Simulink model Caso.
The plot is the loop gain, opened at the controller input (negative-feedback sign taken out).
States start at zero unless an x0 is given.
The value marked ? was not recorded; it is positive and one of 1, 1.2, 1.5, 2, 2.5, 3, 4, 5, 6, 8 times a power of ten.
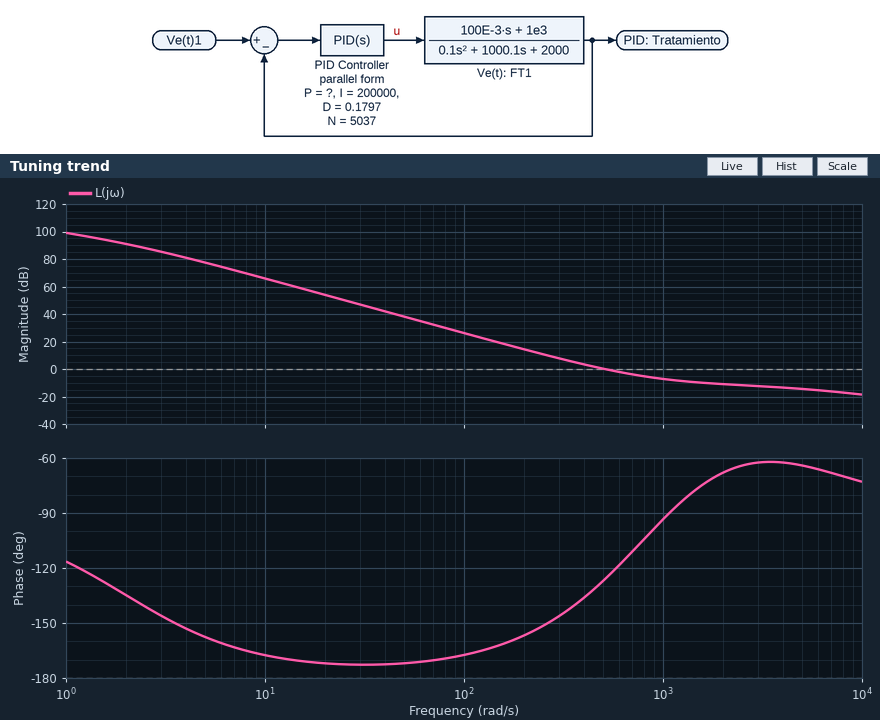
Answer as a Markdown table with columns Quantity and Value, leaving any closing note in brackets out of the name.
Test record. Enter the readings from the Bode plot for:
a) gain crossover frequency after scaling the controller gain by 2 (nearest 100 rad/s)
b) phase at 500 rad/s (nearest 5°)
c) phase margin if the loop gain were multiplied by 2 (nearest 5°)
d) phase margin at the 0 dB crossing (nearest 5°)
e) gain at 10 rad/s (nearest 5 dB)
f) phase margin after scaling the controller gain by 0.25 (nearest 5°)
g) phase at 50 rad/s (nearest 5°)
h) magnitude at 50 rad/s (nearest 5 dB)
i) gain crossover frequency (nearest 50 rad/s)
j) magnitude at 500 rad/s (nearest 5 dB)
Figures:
| Quantity | Value |
|---|---|
| gain crossover frequency after scaling the controller gain by 2 | 900 rad/s |
| phase at 500 rad/s | -125° |
| phase margin if the loop gain were multiplied by 2 | 80° |
| phase margin at the 0 dB crossing | 55° |
| gain at 10 rad/s | 65 dB |
| phase margin after scaling the controller gain by 0.25 | 25° |
| phase at 50 rad/s | -170° |
| magnitude at 50 rad/s | 40 dB |
| gain crossover frequency | 500 rad/s |
| magnitude at 500 rad/s | 0 dB |
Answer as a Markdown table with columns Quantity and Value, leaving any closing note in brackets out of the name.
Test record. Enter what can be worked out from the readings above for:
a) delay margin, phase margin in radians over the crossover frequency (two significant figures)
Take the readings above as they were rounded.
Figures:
| Quantity | Value |
|---|---|
| delay margin, phase margin in radians over the crossover frequency | 0.0019 s |
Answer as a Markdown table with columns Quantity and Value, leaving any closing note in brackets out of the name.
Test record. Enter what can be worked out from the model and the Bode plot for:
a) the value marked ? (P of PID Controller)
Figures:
| Quantity | Value |
|---|---|
| the value marked ? | 400 |
